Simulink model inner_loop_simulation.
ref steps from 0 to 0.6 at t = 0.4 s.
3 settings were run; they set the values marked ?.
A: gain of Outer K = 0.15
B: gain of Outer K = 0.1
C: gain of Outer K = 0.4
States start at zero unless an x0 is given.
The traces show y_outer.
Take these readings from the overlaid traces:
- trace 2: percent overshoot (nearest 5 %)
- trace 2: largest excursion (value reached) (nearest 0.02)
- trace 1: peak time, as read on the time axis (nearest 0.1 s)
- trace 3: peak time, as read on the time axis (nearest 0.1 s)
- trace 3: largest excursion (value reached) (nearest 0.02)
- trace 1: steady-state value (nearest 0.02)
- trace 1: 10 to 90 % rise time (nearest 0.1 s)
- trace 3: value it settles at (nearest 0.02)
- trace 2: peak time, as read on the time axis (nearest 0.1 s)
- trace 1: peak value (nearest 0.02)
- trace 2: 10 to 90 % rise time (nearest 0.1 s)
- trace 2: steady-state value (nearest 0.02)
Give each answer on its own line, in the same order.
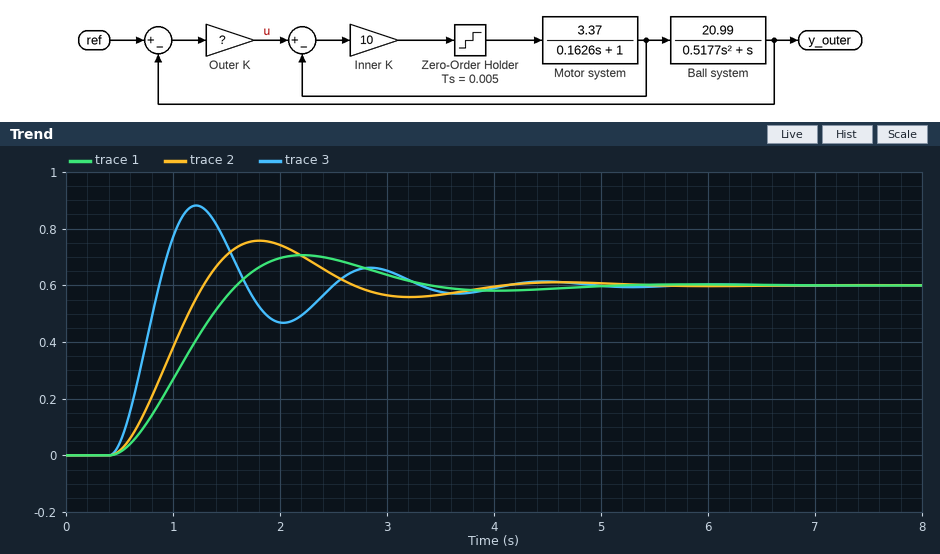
25 %
0.76
2.2 s
1.2 s
0.88
0.60
0.8 s
0.60
1.8 s
0.70
0.6 s
0.60
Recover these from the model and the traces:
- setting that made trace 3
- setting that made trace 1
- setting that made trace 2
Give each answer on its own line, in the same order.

C
B
A
